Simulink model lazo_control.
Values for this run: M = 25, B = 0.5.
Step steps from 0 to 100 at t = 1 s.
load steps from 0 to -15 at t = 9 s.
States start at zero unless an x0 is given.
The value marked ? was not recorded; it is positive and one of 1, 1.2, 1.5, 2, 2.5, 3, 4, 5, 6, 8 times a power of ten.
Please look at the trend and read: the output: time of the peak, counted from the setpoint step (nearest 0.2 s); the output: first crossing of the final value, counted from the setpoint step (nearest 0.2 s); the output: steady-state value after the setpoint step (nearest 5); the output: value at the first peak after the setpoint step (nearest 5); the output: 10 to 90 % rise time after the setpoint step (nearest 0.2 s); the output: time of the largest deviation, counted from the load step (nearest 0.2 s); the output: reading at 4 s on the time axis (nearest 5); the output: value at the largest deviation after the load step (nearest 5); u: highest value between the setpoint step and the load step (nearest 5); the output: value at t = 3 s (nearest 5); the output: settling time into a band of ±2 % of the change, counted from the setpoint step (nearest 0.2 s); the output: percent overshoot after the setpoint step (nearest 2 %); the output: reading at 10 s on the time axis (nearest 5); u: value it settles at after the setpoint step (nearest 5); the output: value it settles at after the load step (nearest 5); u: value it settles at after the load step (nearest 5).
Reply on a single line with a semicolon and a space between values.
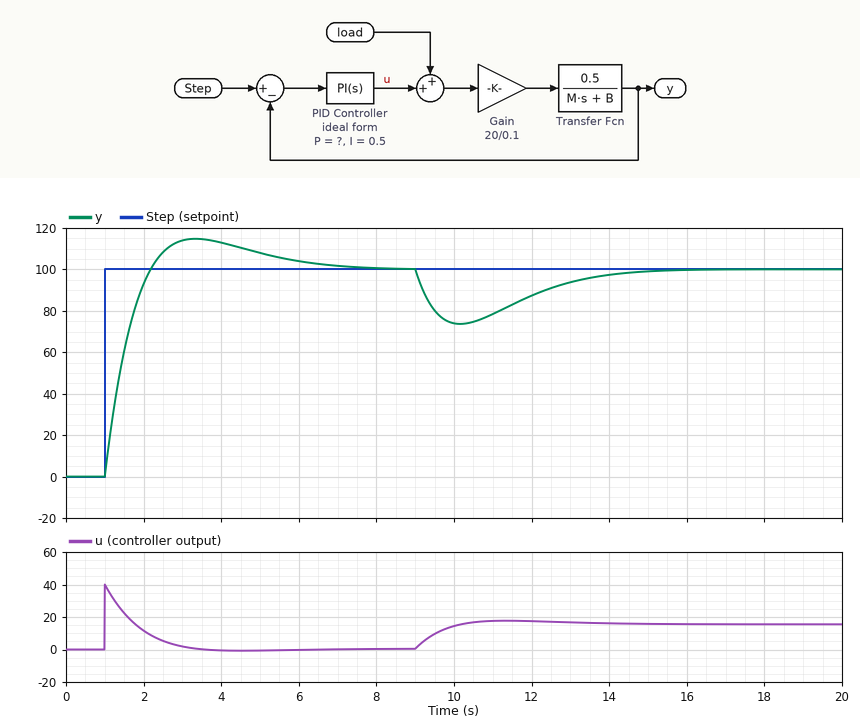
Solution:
2.4 s; 1.2 s; 100; 115; 0.8 s; 1.2 s; 115; 75; 40; 115; 5.8 s; 14 %; 75; 0; 100; 15
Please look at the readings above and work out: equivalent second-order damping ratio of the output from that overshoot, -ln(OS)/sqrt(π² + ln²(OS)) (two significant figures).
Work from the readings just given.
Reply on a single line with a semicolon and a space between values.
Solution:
0.53
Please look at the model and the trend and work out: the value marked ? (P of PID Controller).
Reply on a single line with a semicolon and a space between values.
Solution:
0.4
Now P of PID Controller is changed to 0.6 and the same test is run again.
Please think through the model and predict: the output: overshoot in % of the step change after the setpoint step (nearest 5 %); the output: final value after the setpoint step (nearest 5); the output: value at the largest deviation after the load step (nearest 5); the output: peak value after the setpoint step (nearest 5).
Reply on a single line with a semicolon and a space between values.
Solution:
10 %; 100; 80; 110
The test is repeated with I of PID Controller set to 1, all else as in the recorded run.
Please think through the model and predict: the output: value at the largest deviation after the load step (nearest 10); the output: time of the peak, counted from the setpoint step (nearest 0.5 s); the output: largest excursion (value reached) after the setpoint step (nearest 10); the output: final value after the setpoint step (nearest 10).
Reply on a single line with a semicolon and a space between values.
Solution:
80; 2.0 s; 120; 100
